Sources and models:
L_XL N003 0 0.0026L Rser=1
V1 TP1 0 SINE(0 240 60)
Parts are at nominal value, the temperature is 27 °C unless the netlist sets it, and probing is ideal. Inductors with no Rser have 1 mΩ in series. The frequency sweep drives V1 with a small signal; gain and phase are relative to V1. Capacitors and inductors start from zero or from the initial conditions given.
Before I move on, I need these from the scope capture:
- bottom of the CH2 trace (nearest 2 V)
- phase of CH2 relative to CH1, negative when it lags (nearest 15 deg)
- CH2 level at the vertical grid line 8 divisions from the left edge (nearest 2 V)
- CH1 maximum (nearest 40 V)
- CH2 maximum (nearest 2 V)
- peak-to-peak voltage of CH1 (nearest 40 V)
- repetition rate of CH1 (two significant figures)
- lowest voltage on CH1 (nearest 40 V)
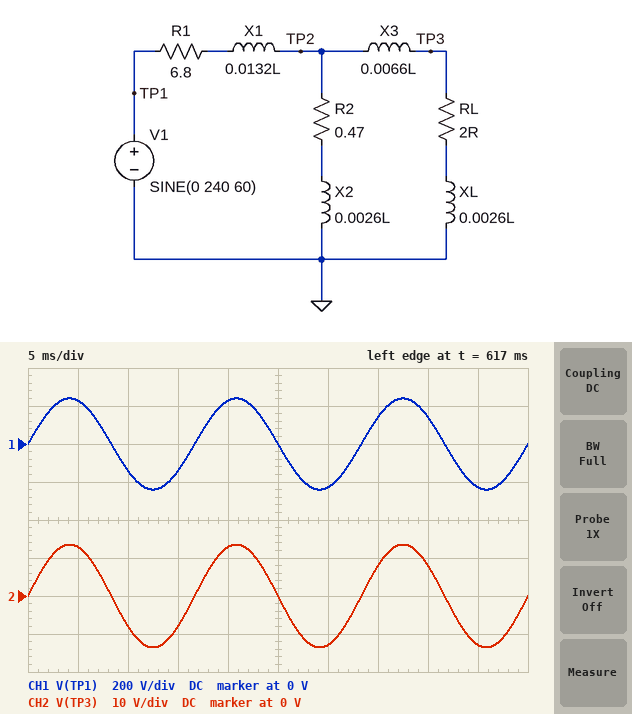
-14 V
0 deg
8 V
240 V
14 V
480 V
60 Hz
-240 V
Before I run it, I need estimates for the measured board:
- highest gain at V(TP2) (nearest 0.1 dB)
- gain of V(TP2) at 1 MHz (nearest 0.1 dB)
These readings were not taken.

-17.5 dB
-17.5 dB
